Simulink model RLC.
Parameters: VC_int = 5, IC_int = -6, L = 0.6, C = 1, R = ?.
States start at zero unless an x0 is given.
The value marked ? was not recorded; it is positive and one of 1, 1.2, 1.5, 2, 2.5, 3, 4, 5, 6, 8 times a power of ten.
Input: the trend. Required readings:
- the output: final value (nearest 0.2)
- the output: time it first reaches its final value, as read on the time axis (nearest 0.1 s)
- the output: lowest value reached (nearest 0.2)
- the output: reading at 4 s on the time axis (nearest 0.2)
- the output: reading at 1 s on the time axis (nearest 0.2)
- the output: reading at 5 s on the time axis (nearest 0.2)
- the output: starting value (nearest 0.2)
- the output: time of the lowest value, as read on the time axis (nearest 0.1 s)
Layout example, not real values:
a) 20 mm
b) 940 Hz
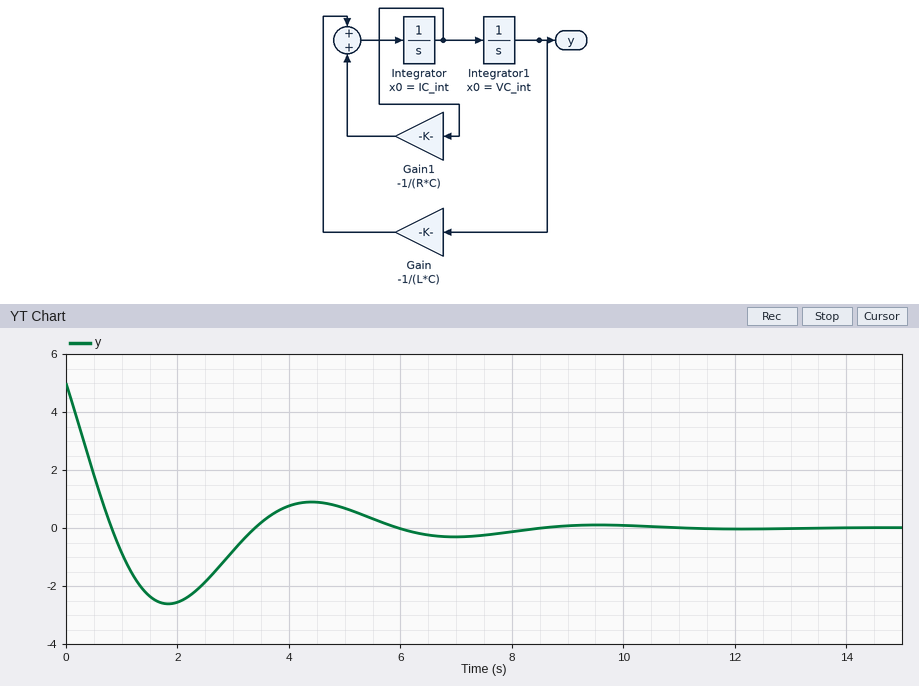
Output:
a) 0.0
b) 0.8 s
c) -2.6
d) 0.8
e) -0.8
f) 0.6
g) 5.0
h) 1.8 s
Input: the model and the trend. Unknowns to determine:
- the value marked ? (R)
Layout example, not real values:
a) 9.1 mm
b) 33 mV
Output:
a) 1.2
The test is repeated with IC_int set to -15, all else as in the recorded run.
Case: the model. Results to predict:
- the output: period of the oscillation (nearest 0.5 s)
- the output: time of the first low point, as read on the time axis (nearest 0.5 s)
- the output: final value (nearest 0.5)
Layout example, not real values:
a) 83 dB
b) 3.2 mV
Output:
a) 5.0 s
b) 1.5 s
c) 0.0
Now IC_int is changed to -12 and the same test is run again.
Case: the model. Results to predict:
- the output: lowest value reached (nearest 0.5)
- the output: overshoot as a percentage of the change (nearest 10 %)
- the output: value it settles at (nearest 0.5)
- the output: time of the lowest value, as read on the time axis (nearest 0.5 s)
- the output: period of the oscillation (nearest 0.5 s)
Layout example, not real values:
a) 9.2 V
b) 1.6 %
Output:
a) -5.0
b) 100 %
c) 0.0
d) 1.5 s
e) 5.0 s
